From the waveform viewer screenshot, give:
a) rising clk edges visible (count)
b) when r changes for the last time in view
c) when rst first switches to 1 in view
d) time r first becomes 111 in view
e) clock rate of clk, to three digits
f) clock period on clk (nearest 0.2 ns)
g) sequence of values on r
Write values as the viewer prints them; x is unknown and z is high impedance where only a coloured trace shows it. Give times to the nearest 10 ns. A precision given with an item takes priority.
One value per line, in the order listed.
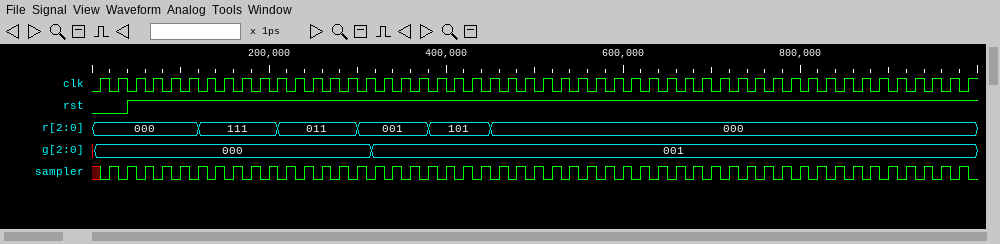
50
450 ns
40 ns
120 ns
50.0 MHz
20 ns
000, 111, 011, 001, 101, 000
